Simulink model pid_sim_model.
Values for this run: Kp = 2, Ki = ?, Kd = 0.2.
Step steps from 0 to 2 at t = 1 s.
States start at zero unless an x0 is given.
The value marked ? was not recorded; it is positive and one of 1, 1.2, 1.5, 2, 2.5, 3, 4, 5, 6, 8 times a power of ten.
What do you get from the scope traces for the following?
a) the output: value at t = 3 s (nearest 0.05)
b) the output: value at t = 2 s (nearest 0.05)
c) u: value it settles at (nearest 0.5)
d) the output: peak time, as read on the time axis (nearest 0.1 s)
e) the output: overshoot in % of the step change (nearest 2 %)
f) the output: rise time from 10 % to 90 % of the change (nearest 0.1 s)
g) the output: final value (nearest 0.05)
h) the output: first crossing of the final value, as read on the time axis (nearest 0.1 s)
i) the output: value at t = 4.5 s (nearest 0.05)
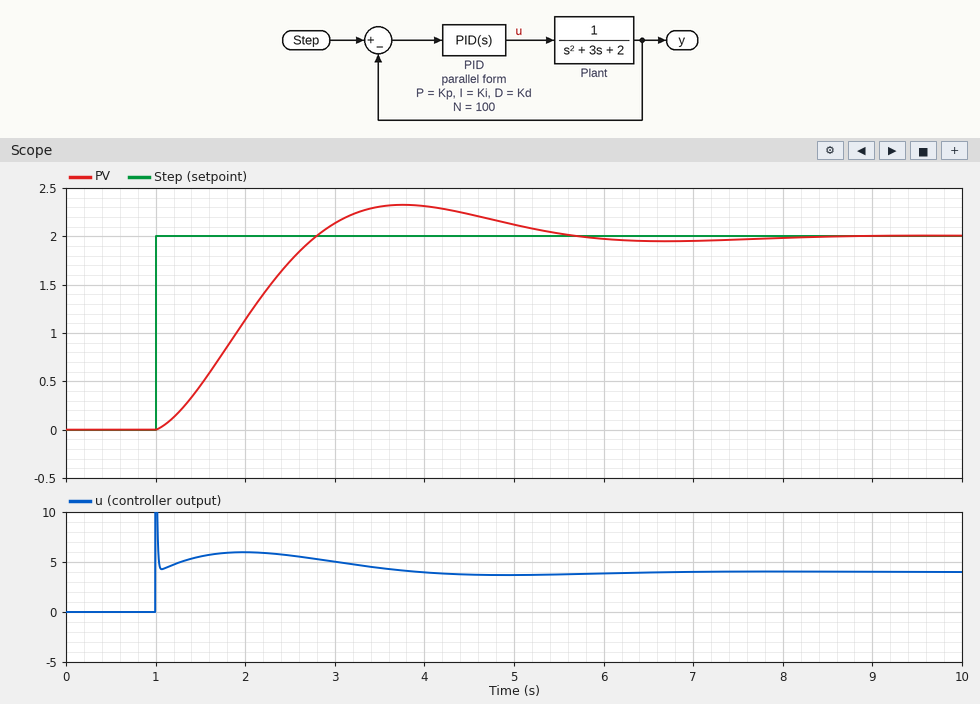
2.15
1.15
4.0
3.8 s
16 %
1.3 s
2.00
2.8 s
2.25
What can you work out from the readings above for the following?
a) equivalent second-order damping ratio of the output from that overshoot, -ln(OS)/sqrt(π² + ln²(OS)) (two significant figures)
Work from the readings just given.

0.50
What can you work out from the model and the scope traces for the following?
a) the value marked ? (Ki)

3
